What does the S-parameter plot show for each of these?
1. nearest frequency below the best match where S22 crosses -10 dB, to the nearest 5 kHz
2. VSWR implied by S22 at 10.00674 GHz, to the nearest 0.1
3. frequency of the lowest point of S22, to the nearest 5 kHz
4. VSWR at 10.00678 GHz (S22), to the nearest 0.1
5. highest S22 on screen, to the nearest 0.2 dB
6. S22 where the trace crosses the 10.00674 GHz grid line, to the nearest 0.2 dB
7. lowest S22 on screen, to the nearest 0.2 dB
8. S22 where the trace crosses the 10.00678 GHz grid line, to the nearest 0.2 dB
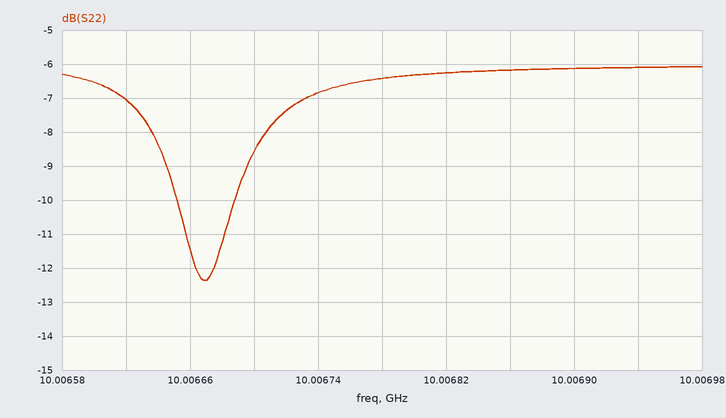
10.006650 GHz
2.7
10.006670 GHz
2.8
-6.0 dB
-6.8 dB
-12.4 dB
-6.4 dB
